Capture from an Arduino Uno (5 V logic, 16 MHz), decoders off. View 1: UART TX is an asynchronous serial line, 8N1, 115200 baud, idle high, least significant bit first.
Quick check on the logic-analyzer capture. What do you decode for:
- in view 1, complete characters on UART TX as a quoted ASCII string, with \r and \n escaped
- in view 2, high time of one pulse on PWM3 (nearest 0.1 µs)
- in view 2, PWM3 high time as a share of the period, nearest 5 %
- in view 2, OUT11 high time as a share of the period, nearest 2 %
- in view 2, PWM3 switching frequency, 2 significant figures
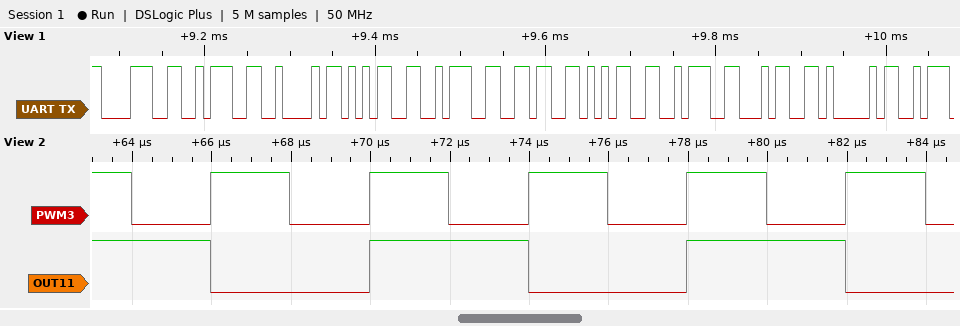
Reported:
"8:B5:65:4A"
2.0 µs
50 %
50 %
250 kHz
